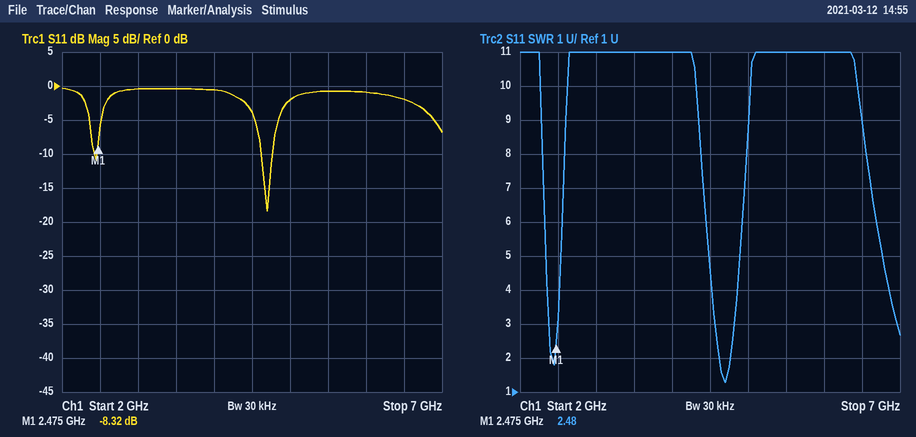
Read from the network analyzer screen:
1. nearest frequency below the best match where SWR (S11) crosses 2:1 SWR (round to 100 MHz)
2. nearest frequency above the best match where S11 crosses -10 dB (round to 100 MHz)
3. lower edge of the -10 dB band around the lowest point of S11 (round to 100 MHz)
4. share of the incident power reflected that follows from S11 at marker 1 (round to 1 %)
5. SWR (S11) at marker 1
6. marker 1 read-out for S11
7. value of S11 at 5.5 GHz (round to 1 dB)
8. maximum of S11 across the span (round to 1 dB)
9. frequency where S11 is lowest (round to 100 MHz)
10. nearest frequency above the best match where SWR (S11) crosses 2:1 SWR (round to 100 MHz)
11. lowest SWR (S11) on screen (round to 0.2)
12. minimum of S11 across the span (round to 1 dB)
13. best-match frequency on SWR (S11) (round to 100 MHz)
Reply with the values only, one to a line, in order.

4.6 GHz
4.8 GHz
4.6 GHz
15 %
2.48
-8.32 dB
-1 dB
0 dB
4.7 GHz
4.8 GHz
1.2
-18 dB
4.7 GHz
